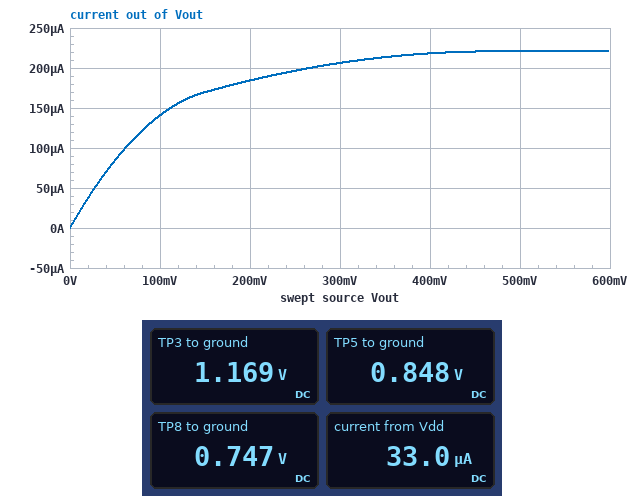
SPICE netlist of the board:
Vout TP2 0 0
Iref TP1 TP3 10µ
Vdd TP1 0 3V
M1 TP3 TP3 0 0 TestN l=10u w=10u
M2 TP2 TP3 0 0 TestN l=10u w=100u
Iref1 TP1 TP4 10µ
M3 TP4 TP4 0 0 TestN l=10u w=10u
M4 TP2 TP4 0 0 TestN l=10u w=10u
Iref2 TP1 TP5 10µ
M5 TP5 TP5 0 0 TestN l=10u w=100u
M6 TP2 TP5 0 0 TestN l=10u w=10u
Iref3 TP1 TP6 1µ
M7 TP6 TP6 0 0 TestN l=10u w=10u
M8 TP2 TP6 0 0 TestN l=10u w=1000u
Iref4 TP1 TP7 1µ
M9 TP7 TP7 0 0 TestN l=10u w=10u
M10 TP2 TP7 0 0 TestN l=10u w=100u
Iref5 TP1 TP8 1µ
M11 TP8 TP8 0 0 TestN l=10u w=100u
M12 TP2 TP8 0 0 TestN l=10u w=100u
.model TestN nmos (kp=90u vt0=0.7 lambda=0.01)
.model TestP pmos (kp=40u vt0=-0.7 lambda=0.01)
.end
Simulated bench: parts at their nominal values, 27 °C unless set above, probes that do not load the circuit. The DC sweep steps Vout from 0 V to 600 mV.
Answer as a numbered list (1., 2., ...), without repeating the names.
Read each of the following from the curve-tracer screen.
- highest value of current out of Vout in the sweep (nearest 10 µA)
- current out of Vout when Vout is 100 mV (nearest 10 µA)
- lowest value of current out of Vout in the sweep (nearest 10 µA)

1. 220 µA
2. 140 µA
3. 0 A
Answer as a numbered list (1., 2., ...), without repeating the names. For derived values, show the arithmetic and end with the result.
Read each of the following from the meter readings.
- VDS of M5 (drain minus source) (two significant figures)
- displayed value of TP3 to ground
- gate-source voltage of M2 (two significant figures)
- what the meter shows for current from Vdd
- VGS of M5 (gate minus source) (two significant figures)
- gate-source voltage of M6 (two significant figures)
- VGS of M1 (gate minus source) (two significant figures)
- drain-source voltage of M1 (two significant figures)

1. 848 mV = 850 mV
2. 1.169 V
3. 1.169 V = 1.2 V
4. 33.0 µA
5. 848 mV = 850 mV
6. 848 mV = 850 mV
7. 1.169 V = 1.2 V
8. 1.169 V = 1.2 V
